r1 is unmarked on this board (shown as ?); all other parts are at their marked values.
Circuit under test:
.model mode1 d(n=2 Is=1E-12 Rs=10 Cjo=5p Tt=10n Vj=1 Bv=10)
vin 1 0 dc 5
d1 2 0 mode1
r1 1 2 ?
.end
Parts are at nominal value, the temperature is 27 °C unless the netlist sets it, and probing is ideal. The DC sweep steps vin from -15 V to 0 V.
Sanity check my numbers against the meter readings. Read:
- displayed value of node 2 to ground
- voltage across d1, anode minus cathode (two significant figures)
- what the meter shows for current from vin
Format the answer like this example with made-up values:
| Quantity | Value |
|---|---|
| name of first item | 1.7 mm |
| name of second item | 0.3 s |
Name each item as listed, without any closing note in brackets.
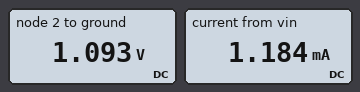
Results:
| Quantity | Value |
|---|---|
| displayed value of node 2 to ground | 1.093 V |
| voltage across d1, anode minus cathode | 1.1 V |
| what the meter shows for current from vin | 1.184 mA |
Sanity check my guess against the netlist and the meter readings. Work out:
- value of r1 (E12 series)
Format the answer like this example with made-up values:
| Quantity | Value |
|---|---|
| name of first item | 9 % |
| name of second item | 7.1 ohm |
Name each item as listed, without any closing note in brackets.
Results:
| Quantity | Value |
|---|---|
| value of r1 | 3.3 kΩ |
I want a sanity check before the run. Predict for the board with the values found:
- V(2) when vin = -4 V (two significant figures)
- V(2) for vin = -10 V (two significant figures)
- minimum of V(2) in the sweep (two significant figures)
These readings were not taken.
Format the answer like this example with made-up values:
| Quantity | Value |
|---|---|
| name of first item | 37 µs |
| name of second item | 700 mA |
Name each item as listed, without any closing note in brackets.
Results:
| Quantity | Value |
|---|---|
| V(2) when vin = -4 V | -4.0 V |
| V(2) for vin = -10 V | -9.8 V |
| minimum of V(2) in the sweep | -10 V |
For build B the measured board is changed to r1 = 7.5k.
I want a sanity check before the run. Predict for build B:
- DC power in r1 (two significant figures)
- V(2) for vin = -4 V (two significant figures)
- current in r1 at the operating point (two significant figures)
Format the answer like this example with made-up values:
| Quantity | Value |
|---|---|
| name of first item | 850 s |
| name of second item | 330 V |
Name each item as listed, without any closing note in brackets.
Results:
| Quantity | Value |
|---|---|
| DC power in r1 | 2.1 mW |
| V(2) for vin = -4 V | -4.0 V |
| current in r1 at the operating point | 530 µA |
